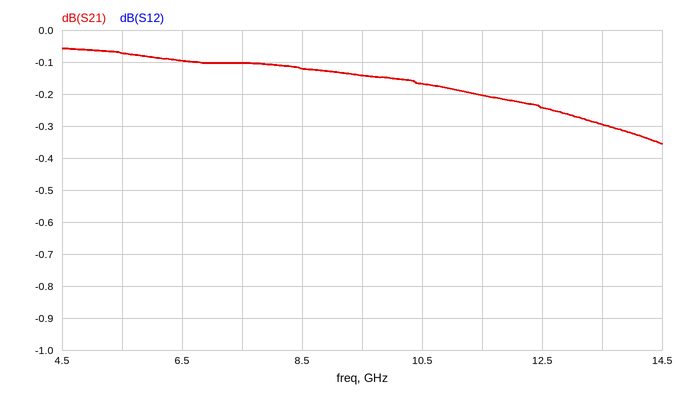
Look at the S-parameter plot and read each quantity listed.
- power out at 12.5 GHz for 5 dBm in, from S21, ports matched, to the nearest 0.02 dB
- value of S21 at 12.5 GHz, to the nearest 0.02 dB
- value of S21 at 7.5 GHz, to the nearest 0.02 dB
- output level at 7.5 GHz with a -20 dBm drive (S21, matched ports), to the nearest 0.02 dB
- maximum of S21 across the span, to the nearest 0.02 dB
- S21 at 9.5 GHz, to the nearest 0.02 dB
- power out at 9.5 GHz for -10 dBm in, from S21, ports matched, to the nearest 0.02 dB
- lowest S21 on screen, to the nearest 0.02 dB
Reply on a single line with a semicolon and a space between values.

4.76 dBm; -0.24 dB; -0.10 dB; -20.10 dBm; -0.06 dB; -0.14 dB; -10.14 dBm; -0.36 dB
